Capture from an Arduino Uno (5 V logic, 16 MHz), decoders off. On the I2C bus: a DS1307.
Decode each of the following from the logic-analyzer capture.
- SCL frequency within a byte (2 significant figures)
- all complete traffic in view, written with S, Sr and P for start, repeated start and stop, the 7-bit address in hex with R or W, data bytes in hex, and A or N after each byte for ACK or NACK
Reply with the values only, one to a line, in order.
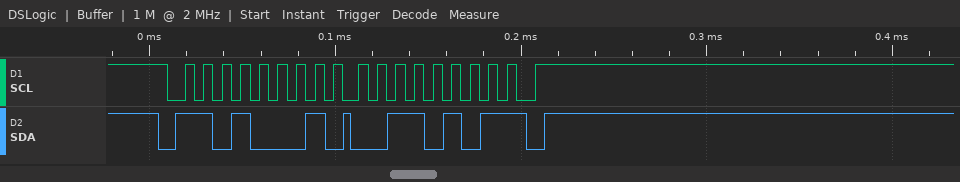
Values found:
100 kHz
S 68R A 35 N P
